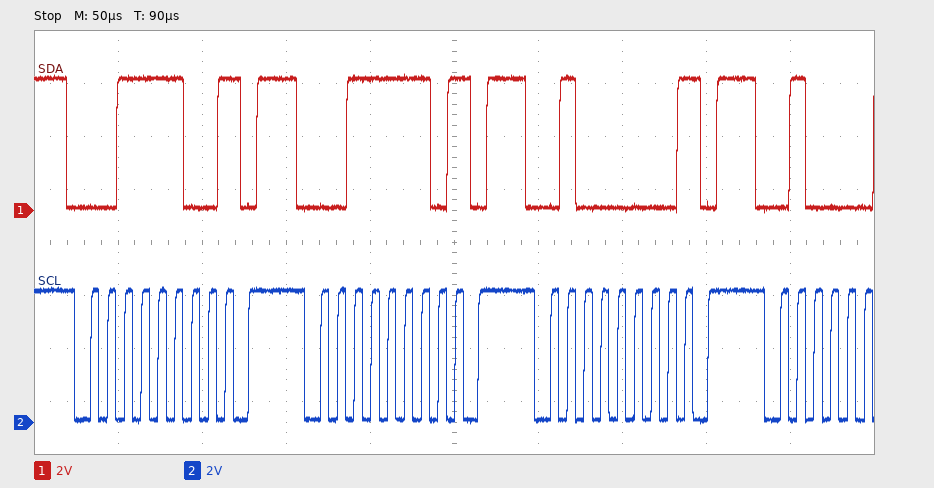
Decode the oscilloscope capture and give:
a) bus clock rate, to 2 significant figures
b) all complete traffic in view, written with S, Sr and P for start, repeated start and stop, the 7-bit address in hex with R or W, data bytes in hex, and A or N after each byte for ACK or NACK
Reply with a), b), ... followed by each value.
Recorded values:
a) 100 kHz
b) S 1EW N P S 1FW N P S 20W N P
